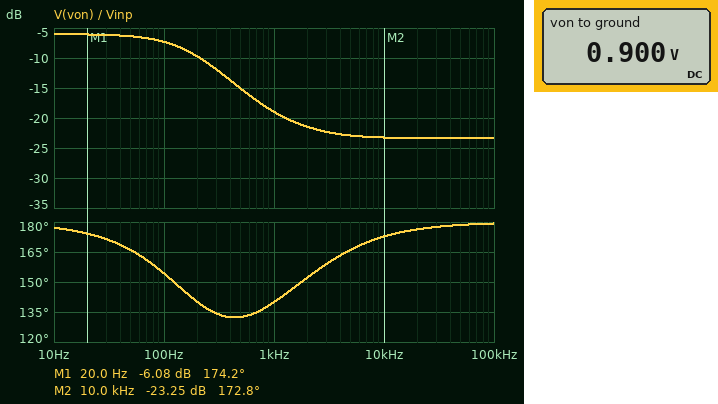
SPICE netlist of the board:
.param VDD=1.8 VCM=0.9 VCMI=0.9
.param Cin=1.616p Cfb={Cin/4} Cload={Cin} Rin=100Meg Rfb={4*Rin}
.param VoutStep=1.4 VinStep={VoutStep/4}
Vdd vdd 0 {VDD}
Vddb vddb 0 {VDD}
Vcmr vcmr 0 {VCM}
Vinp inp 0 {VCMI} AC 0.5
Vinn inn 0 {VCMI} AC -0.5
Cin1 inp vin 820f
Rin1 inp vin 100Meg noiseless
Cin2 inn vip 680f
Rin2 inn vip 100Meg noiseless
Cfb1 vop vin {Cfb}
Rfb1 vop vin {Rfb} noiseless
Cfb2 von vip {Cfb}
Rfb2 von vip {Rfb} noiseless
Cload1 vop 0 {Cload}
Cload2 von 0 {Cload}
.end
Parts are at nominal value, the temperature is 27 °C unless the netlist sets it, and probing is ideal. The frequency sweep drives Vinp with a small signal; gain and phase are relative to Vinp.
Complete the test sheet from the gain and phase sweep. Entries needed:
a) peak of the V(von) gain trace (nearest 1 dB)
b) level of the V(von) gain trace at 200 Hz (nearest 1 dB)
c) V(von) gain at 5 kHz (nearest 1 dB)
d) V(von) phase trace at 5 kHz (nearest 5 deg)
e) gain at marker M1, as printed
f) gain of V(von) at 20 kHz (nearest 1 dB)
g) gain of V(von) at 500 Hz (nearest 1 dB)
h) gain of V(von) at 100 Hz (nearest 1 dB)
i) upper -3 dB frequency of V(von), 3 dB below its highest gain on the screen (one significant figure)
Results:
-6 dB
-10 dB
-23 dB
165 deg
-6.08 dB
-23 dB
-15 dB
-7 dB
200 Hz
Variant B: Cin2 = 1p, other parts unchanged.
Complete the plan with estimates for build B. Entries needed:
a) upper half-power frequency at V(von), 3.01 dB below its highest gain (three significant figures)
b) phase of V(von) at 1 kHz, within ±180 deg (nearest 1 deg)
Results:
171 Hz
142 deg
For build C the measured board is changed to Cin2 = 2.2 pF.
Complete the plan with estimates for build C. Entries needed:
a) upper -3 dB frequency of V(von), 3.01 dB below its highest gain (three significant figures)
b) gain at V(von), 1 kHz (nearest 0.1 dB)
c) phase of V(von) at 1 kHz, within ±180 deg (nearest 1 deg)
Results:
168 Hz
-18.5 dB
146 deg
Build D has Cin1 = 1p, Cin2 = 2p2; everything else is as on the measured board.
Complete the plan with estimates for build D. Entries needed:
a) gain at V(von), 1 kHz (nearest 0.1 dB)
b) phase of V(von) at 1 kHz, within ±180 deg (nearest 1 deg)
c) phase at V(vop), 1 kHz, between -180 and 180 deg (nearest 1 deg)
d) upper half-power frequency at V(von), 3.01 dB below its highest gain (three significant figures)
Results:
-18.5 dB
146 deg
-38 deg
168 Hz
